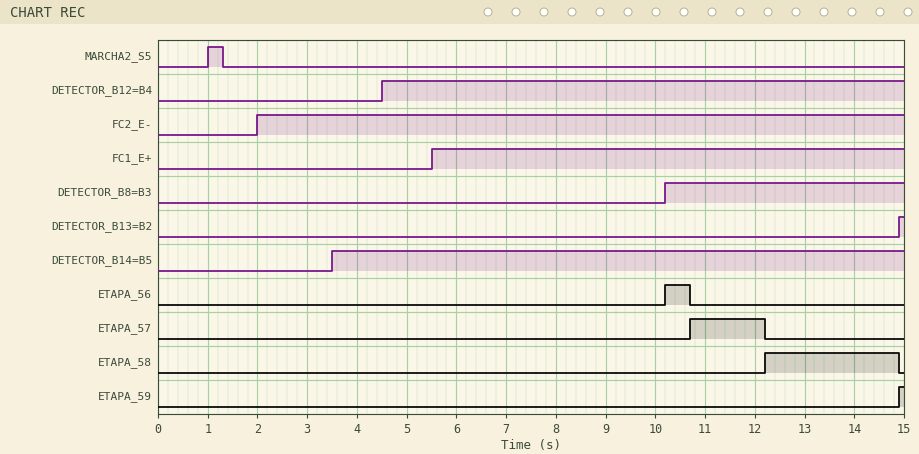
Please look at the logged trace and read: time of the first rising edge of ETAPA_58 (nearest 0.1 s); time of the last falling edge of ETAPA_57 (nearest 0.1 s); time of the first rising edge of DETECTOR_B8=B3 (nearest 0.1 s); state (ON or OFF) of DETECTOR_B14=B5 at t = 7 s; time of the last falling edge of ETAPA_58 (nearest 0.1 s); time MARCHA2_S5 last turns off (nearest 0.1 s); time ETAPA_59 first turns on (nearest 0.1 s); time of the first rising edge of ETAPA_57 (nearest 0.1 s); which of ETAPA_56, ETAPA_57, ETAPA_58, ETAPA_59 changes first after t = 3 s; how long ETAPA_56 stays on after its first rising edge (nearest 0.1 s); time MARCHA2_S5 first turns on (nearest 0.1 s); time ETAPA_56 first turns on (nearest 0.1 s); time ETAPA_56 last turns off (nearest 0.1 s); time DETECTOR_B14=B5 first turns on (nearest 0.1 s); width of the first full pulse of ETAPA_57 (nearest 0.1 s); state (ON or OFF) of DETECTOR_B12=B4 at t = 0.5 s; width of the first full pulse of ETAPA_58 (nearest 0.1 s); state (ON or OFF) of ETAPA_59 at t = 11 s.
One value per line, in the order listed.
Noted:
12.2 s
12.2 s
10.2 s
ON
14.9 s
1.3 s
14.9 s
10.7 s
ETAPA_56
0.5 s
1.0 s
10.2 s
10.7 s
3.5 s
1.5 s
OFF
2.7 s
OFF
